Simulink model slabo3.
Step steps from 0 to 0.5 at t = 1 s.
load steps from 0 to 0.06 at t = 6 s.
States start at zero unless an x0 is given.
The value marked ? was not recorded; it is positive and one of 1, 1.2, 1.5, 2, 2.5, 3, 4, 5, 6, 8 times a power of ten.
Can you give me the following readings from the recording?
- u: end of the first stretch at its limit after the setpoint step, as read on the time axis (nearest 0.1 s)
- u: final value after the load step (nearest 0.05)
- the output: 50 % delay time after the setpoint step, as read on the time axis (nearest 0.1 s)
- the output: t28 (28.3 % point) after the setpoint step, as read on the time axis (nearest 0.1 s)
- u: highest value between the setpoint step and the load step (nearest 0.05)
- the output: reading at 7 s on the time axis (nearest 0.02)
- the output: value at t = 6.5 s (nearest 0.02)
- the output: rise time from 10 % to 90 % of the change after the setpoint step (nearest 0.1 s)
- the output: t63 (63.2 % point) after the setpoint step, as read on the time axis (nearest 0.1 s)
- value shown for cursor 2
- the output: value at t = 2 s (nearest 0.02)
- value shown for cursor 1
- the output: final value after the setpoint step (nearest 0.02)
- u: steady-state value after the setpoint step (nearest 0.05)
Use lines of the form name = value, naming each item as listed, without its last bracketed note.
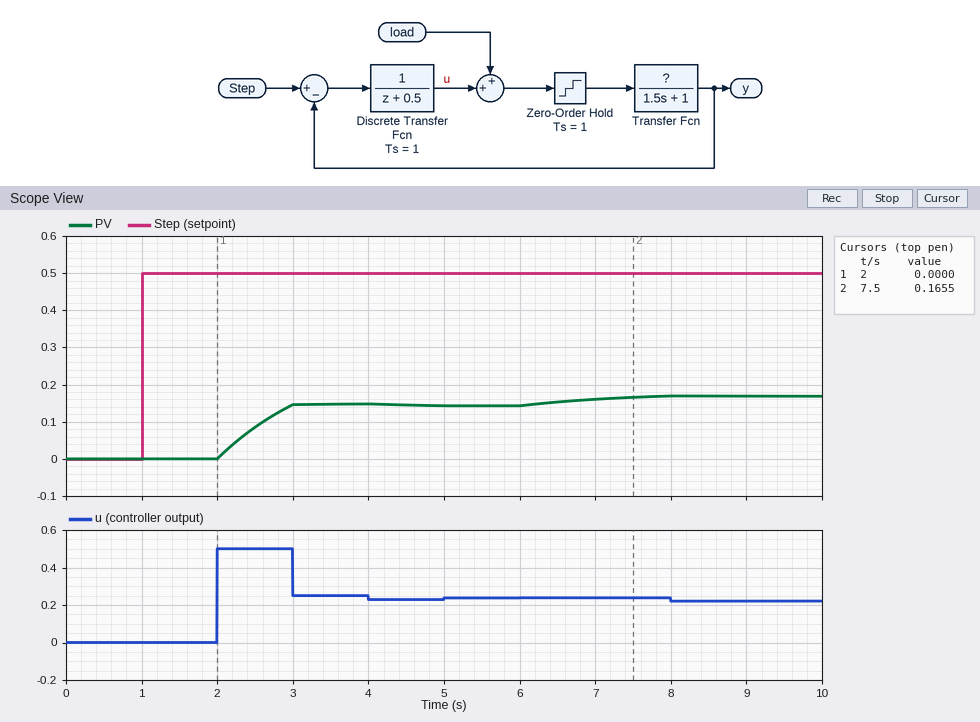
u: end of the first stretch at its limit after the setpoint step, as read on the time axis = 2.0 s
u: final value after the load step = 0.20
the output: 50 % delay time after the setpoint step, as read on the time axis = 2.4 s
the output: t28 (28.3 % point) after the setpoint step, as read on the time axis = 2.2 s
u: highest value between the setpoint step and the load step = 0.50
the output: reading at 7 s on the time axis = 0.16
the output: value at t = 6.5 s = 0.16
the output: rise time from 10 % to 90 % of the change after the setpoint step = 0.8 s
the output: t63 (63.2 % point) after the setpoint step, as read on the time axis = 2.5 s
value shown for cursor 2 = 0.1655
the output: value at t = 2 s = 0.00
value shown for cursor 1 = 0.0000
the output: final value after the setpoint step = 0.14
u: steady-state value after the setpoint step = 0.25
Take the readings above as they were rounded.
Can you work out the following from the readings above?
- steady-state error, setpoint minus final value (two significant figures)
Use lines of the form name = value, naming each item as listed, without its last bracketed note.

steady-state error, setpoint minus final value = 0.36
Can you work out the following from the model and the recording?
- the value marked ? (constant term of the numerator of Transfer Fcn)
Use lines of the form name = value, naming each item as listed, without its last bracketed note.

the value marked ? = 0.6
